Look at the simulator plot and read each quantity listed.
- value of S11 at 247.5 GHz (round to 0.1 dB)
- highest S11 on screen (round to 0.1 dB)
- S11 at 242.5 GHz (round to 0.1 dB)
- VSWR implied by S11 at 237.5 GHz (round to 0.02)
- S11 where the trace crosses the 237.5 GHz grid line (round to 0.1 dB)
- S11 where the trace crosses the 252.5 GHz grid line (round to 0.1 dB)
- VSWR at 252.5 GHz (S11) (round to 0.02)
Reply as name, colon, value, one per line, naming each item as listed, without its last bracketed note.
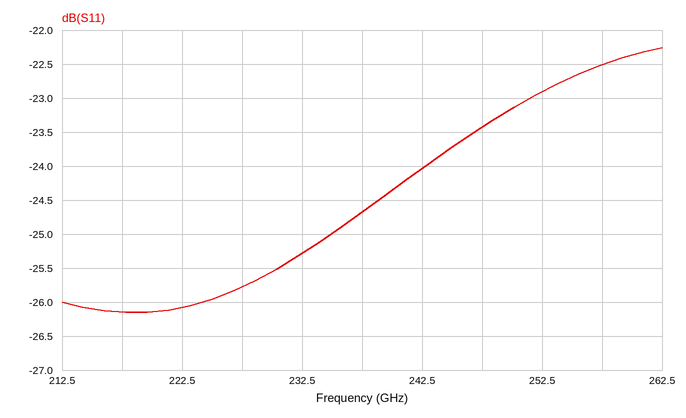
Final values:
value of S11 at 247.5 GHz: -23.4 dB
highest S11 on screen: -22.3 dB
S11 at 242.5 GHz: -24.0 dB
VSWR implied by S11 at 237.5 GHz: 1.12
S11 where the trace crosses the 237.5 GHz grid line: -24.7 dB
S11 where the trace crosses the 252.5 GHz grid line: -22.9 dB
VSWR at 252.5 GHz (S11): 1.16
